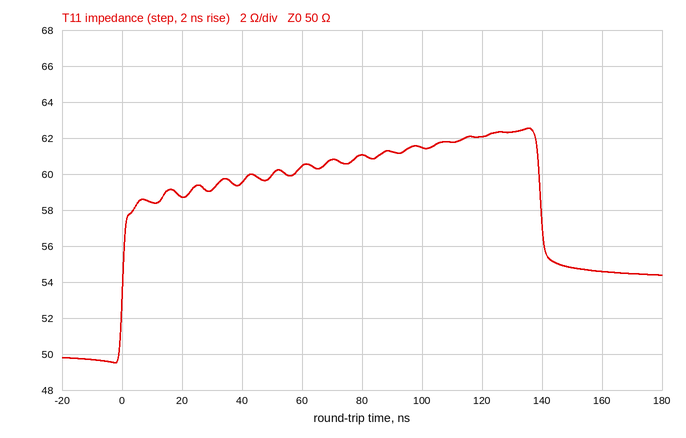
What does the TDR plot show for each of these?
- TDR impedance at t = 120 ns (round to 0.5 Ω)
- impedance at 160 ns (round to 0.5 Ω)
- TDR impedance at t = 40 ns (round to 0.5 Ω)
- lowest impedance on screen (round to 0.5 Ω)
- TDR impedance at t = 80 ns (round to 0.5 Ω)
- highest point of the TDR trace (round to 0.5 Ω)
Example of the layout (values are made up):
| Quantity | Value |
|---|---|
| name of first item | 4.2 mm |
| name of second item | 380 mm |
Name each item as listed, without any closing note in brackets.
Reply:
| Quantity | Value |
|---|---|
| TDR impedance at t = 120 ns | 62.0 Ω |
| impedance at 160 ns | 54.5 Ω |
| TDR impedance at t = 40 ns | 59.5 Ω |
| lowest impedance on screen | 49.5 Ω |
| TDR impedance at t = 80 ns | 61.0 Ω |
| highest point of the TDR trace | 62.5 Ω |
